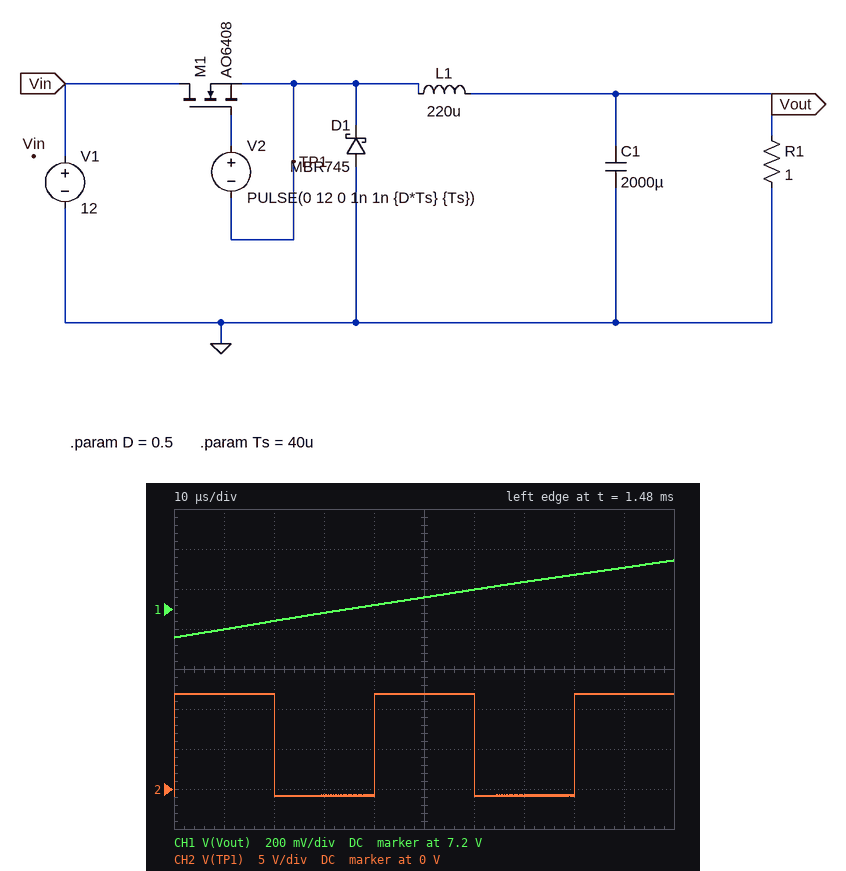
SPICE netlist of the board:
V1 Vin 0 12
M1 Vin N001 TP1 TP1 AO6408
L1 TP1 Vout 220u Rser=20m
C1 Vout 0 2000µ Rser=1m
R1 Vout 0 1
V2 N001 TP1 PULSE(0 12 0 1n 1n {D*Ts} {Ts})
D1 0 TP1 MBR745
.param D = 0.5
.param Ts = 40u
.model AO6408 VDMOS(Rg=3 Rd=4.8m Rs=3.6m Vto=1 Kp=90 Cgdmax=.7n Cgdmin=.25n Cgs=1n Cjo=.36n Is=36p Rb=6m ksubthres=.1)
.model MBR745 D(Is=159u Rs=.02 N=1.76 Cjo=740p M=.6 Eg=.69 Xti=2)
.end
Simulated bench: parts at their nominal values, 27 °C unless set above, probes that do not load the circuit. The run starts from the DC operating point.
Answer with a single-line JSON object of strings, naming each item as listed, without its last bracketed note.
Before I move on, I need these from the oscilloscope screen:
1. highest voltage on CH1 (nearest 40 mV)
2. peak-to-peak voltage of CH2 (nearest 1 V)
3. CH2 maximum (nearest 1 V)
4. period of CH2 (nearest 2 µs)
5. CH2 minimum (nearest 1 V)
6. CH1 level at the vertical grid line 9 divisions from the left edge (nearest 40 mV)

{"highest voltage on CH1": "7.44 V", "peak-to-peak voltage of CH2": "13 V", "CH2 maximum": "12 V", "period of CH2": "40 µs", "CH2 minimum": "-1 V", "CH1 level at the vertical grid line 9 divisions from the left edge": "7.40 V"}
